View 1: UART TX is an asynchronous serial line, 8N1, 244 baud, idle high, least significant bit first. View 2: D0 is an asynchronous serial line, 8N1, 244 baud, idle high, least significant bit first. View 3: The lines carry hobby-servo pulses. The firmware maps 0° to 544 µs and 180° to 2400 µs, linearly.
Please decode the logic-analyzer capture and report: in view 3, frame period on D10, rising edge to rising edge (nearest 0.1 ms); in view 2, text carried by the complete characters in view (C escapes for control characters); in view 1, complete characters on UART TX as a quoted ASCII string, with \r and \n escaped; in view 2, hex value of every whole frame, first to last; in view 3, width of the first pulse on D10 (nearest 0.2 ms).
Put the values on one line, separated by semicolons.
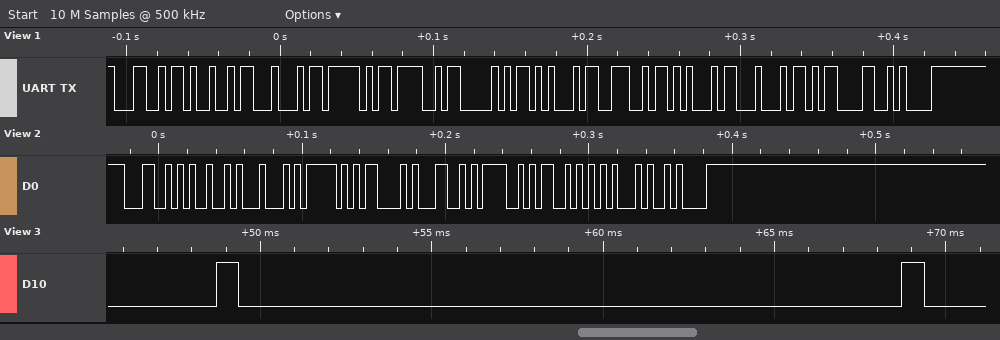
20.0 ms; "LID_CLOSE\n"; "LID_OPENED\r\n"; 4C 49 44 5F 43 4C 4F 53 45 0A; 0.6 ms
